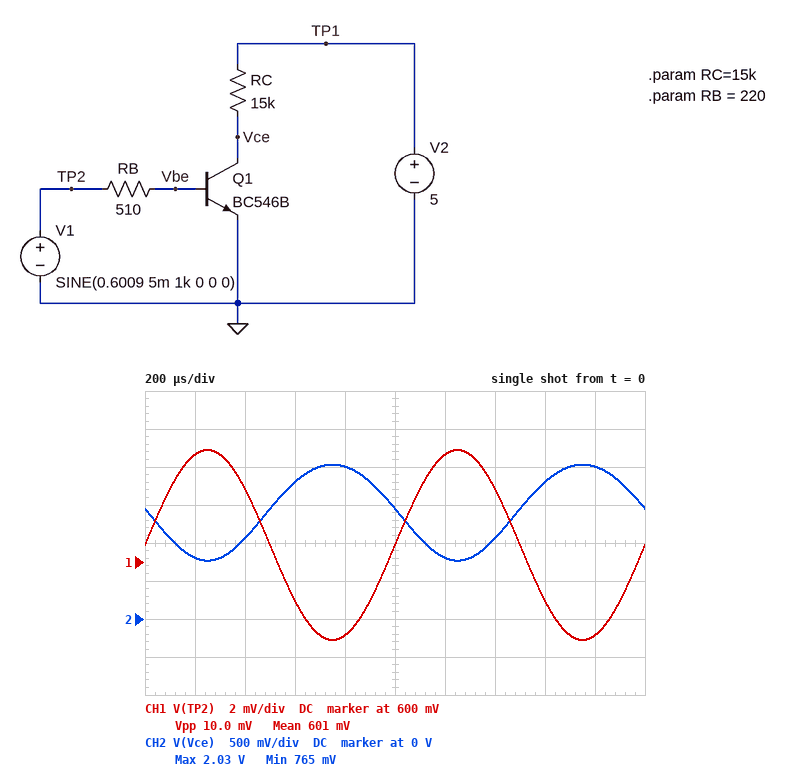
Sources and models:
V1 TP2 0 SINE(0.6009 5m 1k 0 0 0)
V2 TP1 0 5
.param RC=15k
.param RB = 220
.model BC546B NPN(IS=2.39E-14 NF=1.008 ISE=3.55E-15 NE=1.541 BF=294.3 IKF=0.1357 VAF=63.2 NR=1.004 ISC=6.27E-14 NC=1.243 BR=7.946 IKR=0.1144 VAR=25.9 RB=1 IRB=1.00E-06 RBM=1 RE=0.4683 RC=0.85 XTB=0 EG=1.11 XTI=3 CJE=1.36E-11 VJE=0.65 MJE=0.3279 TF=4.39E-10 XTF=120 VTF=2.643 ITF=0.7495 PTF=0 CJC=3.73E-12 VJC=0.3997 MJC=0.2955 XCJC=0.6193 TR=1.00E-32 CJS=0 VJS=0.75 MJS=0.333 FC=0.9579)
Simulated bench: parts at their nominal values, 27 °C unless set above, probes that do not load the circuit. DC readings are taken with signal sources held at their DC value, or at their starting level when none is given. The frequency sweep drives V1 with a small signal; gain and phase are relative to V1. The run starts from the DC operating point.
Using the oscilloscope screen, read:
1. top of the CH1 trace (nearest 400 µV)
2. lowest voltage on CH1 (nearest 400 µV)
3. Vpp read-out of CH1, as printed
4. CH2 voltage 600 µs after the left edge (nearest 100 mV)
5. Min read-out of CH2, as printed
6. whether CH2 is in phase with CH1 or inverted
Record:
606.0 mV
596.0 mV
10.0 mV
1.8 V
765 mV
inverted
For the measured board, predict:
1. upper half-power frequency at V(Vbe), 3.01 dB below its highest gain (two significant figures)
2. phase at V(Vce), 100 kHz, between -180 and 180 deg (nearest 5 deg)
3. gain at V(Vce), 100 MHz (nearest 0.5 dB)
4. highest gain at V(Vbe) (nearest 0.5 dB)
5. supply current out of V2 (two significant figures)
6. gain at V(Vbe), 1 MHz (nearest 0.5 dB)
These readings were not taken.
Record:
730 kHz
170 deg
-7.5 dB
0 dB
240 µA
-4.5 dB
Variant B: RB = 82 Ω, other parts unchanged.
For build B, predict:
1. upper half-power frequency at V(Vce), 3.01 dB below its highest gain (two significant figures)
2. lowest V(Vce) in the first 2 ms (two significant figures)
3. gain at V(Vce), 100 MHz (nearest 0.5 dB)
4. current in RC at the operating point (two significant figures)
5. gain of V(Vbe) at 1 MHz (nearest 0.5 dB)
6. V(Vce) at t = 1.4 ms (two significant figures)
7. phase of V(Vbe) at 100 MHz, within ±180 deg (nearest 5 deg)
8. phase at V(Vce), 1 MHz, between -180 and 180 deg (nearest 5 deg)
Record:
2.3 MHz
700 mV
6.5 dB
240 µA
-0.5 dB
1.0 V
-45 deg
155 deg
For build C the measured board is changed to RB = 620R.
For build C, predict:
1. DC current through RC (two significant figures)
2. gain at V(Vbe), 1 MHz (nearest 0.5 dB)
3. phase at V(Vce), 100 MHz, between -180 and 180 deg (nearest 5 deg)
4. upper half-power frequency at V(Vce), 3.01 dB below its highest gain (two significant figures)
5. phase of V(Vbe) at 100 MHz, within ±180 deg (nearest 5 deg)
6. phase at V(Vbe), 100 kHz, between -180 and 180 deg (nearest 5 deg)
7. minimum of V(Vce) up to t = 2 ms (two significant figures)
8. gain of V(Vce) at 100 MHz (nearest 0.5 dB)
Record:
240 µA
-5.5 dB
15 deg
600 kHz
-65 deg
-10 deg
780 mV
-9.0 dB
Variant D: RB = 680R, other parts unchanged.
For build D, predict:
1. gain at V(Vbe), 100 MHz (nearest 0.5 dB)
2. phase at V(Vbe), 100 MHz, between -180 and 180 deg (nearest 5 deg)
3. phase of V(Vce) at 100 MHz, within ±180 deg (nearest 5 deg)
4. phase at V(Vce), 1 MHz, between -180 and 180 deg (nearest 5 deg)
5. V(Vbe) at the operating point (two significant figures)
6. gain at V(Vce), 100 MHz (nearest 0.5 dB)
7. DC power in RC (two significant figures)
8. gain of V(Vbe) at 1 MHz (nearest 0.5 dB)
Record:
-24.5 dB
-65 deg
15 deg
120 deg
600 mV
-10.0 dB
830 µW
-6.0 dB
